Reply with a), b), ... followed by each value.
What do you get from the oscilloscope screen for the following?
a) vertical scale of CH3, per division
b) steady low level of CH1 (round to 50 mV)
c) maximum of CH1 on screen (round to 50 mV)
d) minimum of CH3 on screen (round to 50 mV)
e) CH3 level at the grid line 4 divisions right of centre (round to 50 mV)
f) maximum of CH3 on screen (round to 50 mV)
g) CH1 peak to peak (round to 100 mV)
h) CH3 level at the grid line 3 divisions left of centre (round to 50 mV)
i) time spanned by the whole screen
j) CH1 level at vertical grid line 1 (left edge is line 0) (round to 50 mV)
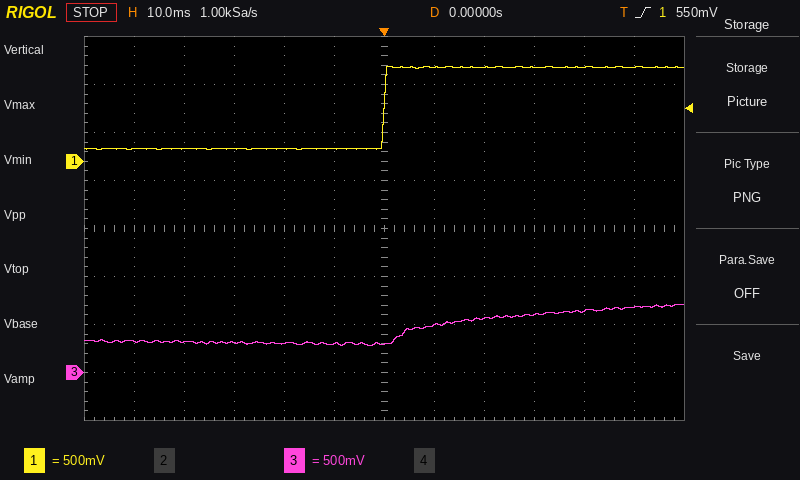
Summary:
a) 500 mV
b) 150 mV
c) 1.00 V
d) 300 mV
e) 650 mV
f) 700 mV
g) 900 mV
h) 300 mV
i) 120 ms
j) 150 mV
